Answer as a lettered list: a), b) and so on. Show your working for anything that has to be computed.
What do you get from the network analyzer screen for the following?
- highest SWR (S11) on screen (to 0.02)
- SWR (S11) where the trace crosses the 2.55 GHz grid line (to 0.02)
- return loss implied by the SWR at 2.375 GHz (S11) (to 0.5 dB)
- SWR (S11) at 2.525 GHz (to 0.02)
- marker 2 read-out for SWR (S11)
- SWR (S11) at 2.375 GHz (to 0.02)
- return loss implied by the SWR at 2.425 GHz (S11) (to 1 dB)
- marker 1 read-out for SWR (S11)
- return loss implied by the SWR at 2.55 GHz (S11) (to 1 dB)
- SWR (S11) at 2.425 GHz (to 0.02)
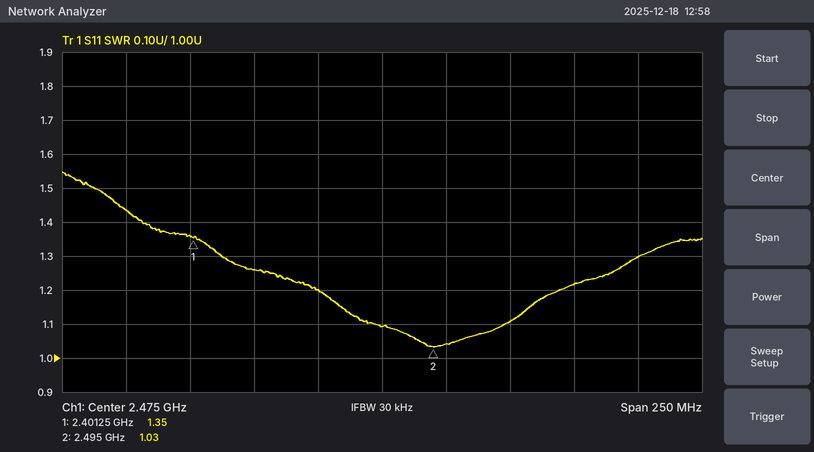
a) 1.54
b) 1.22
c) −20 log10((1.44 − 1)/(1.44 + 1)) ≈ 14.9 dB, so 15.0 dB to the nearest 0.5 dB
d) 1.10
e) 1.03
f) 1.44
g) −20 log10((1.26 − 1)/(1.26 + 1)) ≈ 19 dB
h) 1.35
i) −20 log10((1.22 − 1)/(1.22 + 1)) ≈ 20 dB
j) 1.26
